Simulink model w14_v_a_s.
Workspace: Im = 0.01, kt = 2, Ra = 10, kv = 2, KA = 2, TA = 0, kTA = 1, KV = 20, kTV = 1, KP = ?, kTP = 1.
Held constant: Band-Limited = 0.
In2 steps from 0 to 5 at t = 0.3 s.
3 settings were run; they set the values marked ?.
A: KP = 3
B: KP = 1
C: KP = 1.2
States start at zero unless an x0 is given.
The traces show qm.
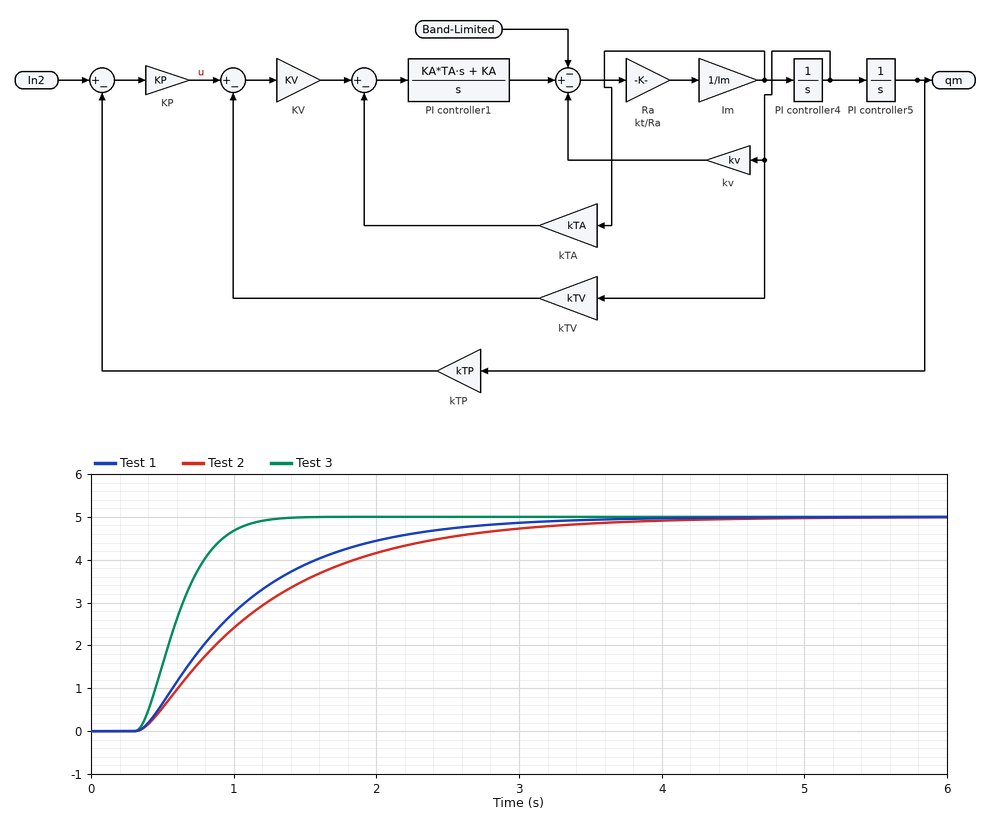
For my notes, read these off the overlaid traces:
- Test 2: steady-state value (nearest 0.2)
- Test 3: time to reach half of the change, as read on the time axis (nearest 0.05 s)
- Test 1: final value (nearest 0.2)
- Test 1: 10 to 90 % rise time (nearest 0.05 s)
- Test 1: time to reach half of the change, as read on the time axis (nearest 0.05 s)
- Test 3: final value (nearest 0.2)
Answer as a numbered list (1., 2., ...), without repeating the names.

1. 5.0
2. 0.60 s
3. 5.0
4. 1.60 s
5. 0.90 s
6. 5.0
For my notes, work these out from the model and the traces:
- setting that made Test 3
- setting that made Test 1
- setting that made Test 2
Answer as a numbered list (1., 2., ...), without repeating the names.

1. A
2. C
3. B
